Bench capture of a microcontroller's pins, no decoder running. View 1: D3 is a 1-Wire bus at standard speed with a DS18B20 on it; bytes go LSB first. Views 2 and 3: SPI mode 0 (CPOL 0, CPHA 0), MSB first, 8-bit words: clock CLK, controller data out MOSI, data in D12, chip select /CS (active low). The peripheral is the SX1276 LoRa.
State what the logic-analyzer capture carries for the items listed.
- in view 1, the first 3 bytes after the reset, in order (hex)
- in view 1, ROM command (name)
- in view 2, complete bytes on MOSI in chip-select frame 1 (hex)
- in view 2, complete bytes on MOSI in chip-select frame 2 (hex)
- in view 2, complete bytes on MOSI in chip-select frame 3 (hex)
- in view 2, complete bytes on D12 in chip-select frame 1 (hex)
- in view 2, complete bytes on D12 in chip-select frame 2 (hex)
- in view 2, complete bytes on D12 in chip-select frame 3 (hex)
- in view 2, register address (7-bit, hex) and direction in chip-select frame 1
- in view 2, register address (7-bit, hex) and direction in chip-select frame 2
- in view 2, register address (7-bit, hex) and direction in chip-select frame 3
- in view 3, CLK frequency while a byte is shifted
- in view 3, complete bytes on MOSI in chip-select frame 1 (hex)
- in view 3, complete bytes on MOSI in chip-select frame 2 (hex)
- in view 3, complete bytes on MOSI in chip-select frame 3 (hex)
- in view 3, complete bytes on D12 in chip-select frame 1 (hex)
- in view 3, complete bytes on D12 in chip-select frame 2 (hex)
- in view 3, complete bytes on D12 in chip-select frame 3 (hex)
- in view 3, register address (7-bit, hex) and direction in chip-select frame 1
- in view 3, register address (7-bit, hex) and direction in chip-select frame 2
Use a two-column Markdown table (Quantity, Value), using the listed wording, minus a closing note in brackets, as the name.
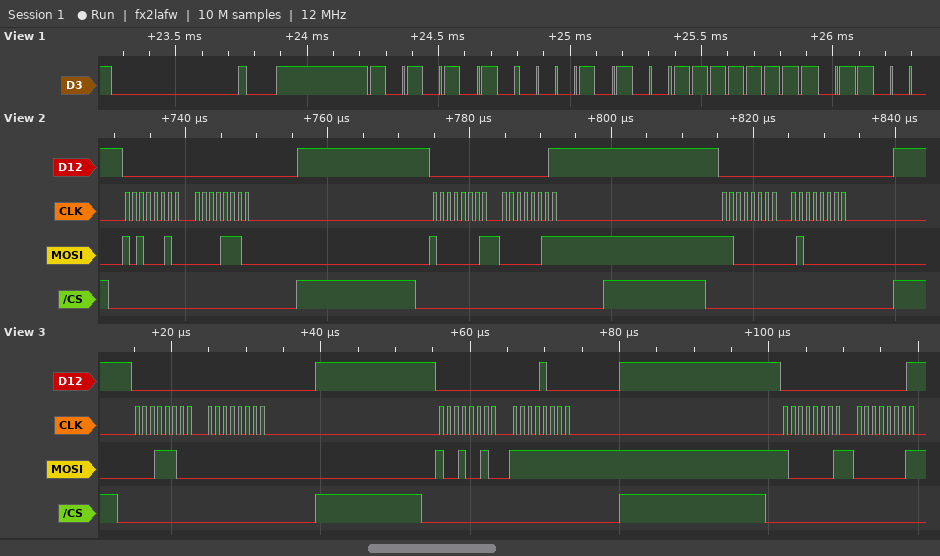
| Quantity | Value |
|---|---|
| in view 1, the first 3 bytes after the reset, in order | 55 28 FF |
| in view 1, ROM command | Match ROM |
| in view 2, complete bytes on MOSI in chip-select frame 1 | 0xA2 0x0E |
| in view 2, complete bytes on MOSI in chip-select frame 2 | 0x81 0x03 |
| in view 2, complete bytes on MOSI in chip-select frame 3 | 0xC0 0x40 |
| in view 2, complete bytes on D12 in chip-select frame 1 | 0x00 0x00 |
| in view 2, complete bytes on D12 in chip-select frame 2 | 0x00 0x01 |
| in view 2, complete bytes on D12 in chip-select frame 3 | 0x00 0x00 |
| in view 2, register address (7-bit, hex) and direction in chip-select frame 1 | 0x22 write |
| in view 2, register address (7-bit, hex) and direction in chip-select frame 2 | 0x01 write |
| in view 2, register address (7-bit, hex) and direction in chip-select frame 3 | 0x40 write |
| in view 3, CLK frequency while a byte is shifted | 1 MHz |
| in view 3, complete bytes on MOSI in chip-select frame 1 | 1C 00 |
| in view 3, complete bytes on MOSI in chip-select frame 2 | 92 FF |
| in view 3, complete bytes on MOSI in chip-select frame 3 | 81 01 |
| in view 3, complete bytes on D12 in chip-select frame 1 | 00 00 |
| in view 3, complete bytes on D12 in chip-select frame 2 | 00 08 |
| in view 3, complete bytes on D12 in chip-select frame 3 | 00 01 |
| in view 3, register address (7-bit, hex) and direction in chip-select frame 1 | 0x1C read |
| in view 3, register address (7-bit, hex) and direction in chip-select frame 2 | 0x12 write |
